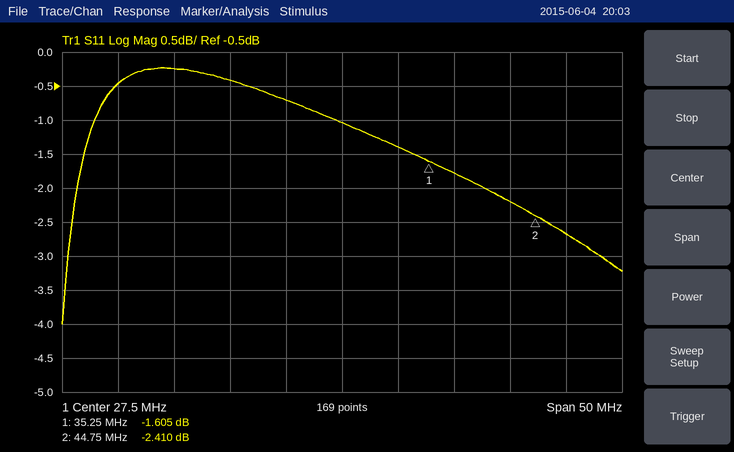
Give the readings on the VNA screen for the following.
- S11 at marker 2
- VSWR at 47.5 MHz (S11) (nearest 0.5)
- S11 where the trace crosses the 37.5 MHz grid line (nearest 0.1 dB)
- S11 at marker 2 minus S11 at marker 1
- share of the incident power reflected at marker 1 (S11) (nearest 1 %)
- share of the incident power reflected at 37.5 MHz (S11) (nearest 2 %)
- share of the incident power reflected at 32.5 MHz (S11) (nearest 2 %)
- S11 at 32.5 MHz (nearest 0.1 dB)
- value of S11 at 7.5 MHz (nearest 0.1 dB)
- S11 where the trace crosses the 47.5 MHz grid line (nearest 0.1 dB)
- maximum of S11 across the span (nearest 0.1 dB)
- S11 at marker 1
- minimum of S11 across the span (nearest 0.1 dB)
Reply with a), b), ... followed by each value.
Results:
a) -2.410 dB
b) 6.5
c) -1.8 dB
d) -0.805 dB
e) 69 %
f) 66 %
g) 72 %
h) -1.4 dB
i) -0.5 dB
j) -2.7 dB
k) -0.2 dB
l) -1.605 dB
m) -4.0 dB
